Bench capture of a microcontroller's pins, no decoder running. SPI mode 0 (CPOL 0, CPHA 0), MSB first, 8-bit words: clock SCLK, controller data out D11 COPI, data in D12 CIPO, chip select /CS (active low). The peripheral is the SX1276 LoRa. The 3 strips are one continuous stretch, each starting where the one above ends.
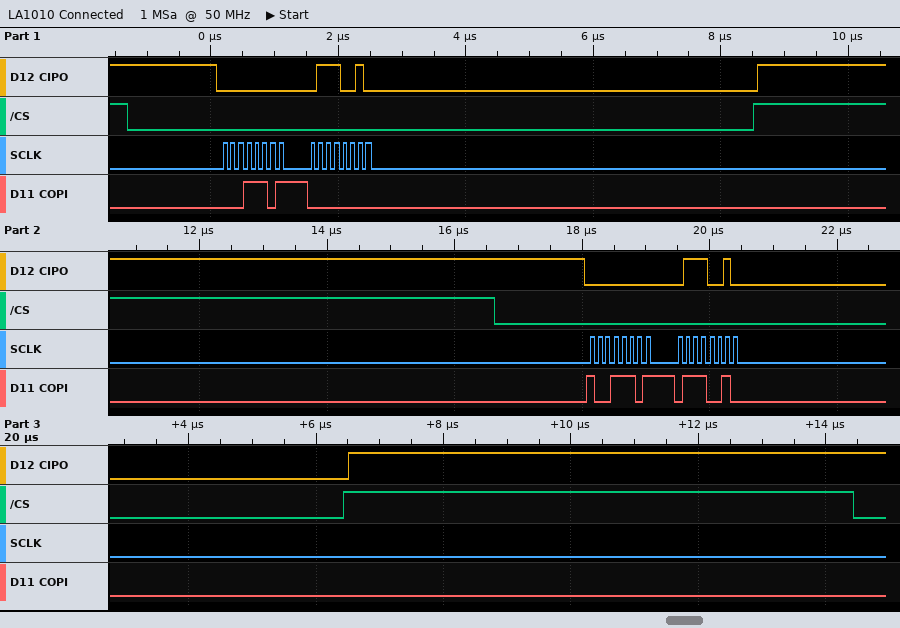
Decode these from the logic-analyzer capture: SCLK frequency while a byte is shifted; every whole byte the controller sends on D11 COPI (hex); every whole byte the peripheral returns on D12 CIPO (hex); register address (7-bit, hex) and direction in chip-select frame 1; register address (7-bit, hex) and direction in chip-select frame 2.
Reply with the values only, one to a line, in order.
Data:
8 MHz
0x1D 0x00 0x9D 0x72
0x00 0x72 0x00 0x72
0x1D read
0x1D write
